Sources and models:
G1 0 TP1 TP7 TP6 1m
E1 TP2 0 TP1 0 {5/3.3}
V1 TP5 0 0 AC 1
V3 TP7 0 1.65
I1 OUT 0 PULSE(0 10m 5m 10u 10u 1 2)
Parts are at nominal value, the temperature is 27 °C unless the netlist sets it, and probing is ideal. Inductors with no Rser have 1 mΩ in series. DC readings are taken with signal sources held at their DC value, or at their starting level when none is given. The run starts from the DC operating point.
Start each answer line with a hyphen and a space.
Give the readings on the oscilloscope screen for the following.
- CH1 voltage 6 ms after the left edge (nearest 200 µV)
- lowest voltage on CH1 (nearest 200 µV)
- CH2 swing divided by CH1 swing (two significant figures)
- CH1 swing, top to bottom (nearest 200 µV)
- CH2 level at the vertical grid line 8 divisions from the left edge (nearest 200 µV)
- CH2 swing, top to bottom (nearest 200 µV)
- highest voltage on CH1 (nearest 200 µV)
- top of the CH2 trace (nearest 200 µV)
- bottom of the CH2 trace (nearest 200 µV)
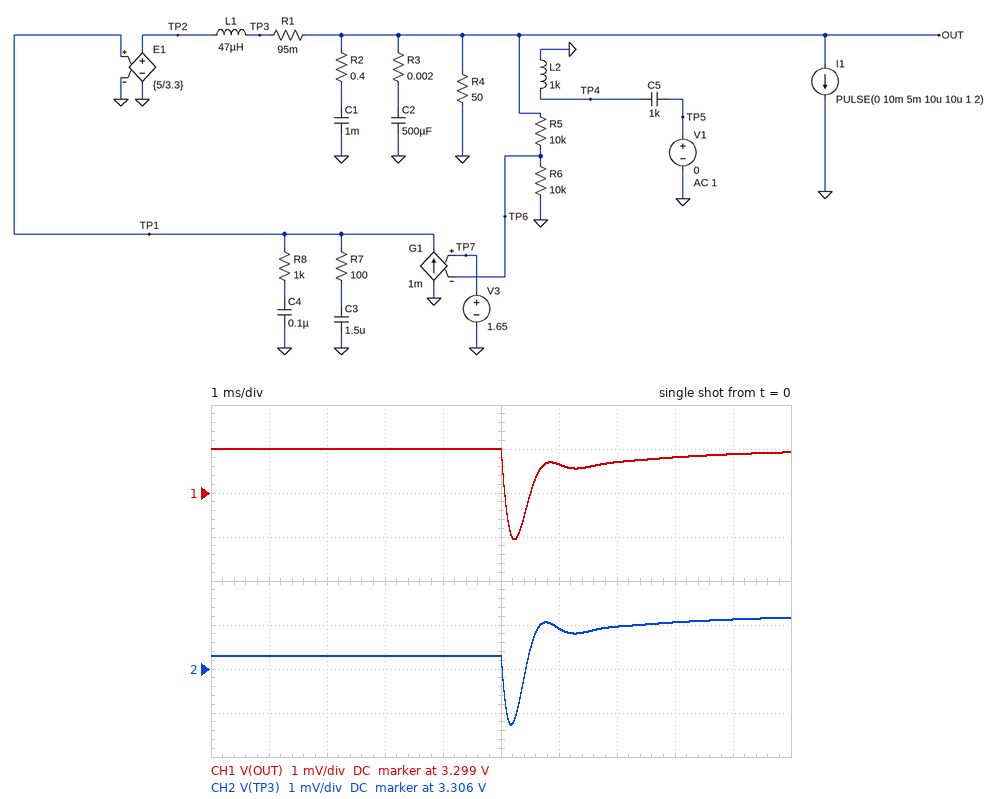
- 3.2996 V
- 3.2980 V
- 1.2
- 2.0 mV
- 3.3070 V
- 2.4 mV
- 3.3000 V
- 3.3072 V
- 3.3048 V
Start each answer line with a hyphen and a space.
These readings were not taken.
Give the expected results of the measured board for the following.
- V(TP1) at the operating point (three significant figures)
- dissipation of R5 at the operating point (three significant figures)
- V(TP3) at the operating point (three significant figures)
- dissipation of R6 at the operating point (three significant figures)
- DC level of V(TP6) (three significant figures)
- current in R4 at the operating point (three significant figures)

- 2.18 V
- 272 µW
- 3.31 V
- 272 µW
- 1.65 V
- 66.0 mA
